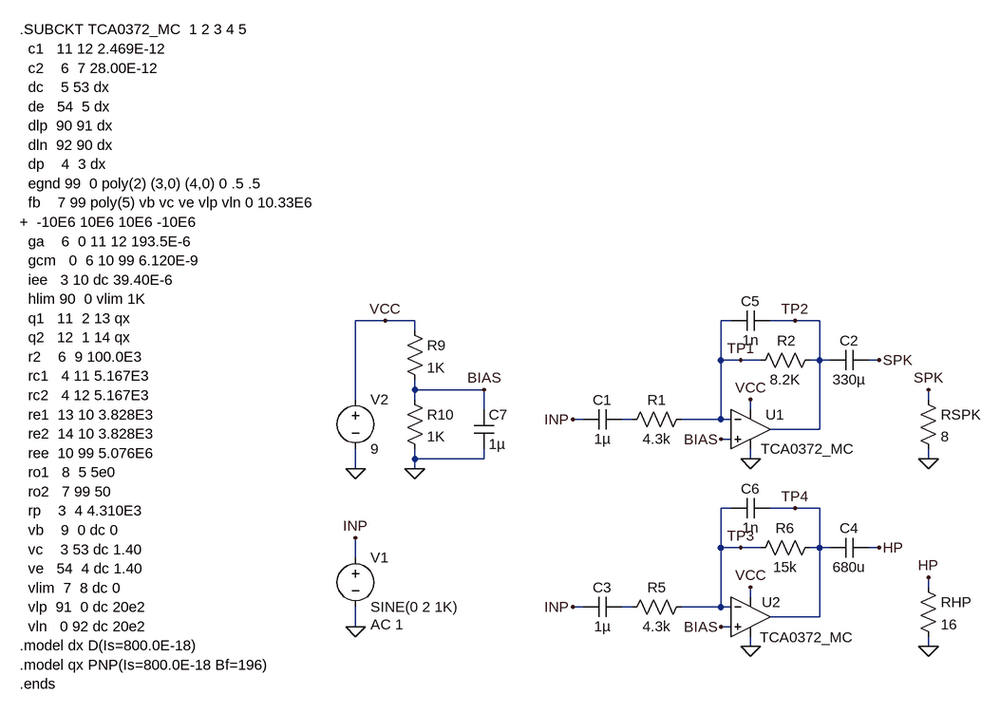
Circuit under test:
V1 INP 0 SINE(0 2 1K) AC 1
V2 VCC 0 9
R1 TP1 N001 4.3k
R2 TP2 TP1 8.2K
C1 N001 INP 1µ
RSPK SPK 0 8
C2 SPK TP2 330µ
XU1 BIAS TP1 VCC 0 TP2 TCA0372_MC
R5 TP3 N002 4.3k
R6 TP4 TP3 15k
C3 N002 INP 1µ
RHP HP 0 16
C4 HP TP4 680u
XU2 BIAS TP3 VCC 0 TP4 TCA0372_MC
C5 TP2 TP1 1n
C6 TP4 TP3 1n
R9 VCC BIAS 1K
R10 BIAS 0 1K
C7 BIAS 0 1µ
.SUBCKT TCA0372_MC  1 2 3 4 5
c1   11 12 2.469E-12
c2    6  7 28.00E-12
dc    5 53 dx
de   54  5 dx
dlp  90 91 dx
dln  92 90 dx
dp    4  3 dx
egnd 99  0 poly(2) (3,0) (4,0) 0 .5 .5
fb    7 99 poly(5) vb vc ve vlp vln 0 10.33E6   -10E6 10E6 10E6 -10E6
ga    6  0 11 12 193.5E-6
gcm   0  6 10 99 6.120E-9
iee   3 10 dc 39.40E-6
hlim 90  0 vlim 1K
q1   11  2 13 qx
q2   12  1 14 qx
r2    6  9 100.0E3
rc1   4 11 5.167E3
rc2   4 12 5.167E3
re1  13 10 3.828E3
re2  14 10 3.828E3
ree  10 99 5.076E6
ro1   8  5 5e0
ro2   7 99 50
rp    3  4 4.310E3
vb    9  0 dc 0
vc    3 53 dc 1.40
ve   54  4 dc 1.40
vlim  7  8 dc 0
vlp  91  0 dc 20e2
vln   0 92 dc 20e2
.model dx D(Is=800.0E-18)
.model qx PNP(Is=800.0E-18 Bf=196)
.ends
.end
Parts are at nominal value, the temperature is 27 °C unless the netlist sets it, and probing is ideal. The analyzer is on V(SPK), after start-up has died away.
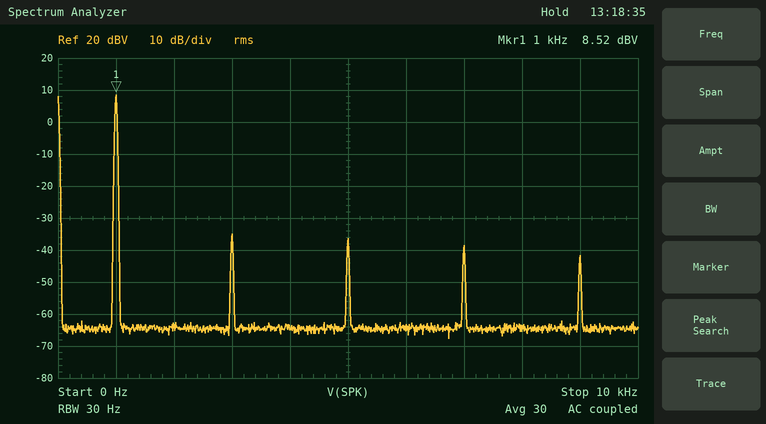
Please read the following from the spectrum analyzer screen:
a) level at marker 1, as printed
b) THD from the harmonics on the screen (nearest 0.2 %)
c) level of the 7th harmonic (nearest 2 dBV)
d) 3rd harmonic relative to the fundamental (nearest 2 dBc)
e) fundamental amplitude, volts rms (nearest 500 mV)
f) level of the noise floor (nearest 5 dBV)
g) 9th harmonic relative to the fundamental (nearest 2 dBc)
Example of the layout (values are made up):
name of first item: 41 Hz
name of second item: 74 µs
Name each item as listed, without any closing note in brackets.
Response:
level at marker 1, as printed: 8.52 dBV
THD from the harmonics on the screen: 1.0 %
level of the 7th harmonic: -38 dBV
3rd harmonic relative to the fundamental: -44 dBc
fundamental amplitude, volts rms: 2.5 V
level of the noise floor: -65 dBV
9th harmonic relative to the fundamental: -50 dBc
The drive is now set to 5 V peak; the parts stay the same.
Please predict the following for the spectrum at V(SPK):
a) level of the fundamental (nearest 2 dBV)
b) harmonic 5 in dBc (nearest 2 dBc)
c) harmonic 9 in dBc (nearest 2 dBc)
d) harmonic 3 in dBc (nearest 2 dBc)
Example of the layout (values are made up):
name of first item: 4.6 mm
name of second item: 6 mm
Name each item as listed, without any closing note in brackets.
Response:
level of the fundamental: 10 dBV
harmonic 5 in dBc: -20 dBc
harmonic 9 in dBc: -38 dBc
harmonic 3 in dBc: -12 dBc
